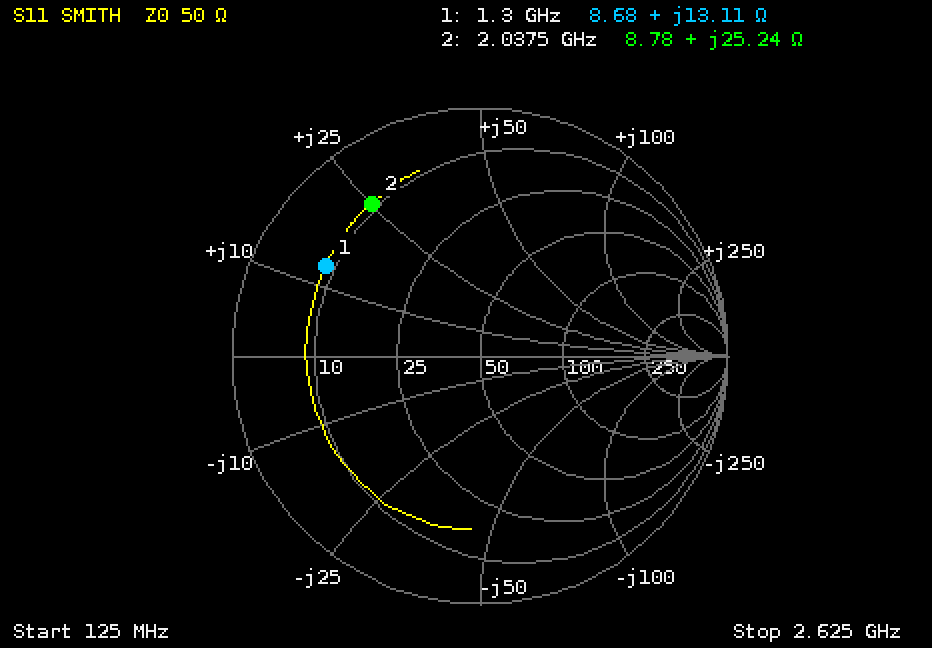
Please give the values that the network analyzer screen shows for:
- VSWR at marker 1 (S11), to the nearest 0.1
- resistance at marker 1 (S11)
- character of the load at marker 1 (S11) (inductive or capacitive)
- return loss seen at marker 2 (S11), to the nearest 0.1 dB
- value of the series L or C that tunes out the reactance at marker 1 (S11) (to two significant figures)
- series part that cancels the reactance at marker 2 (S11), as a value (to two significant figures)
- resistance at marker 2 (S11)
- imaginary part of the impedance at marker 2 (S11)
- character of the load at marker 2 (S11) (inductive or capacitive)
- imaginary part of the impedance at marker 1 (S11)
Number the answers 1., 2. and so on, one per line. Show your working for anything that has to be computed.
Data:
1. 6.2
2. 8.68 Ω
3. inductive
4. 2.4 dB
5. C = 1/(2π × 1.3 GHz × 13.11 Ω) ≈ 9.3 pF
6. C = 1/(2π × 2.0375 GHz × 25.24 Ω) ≈ 3.1 pF
7. 8.78 Ω
8. +25.24 Ω
9. inductive
10. +13.11 Ω
